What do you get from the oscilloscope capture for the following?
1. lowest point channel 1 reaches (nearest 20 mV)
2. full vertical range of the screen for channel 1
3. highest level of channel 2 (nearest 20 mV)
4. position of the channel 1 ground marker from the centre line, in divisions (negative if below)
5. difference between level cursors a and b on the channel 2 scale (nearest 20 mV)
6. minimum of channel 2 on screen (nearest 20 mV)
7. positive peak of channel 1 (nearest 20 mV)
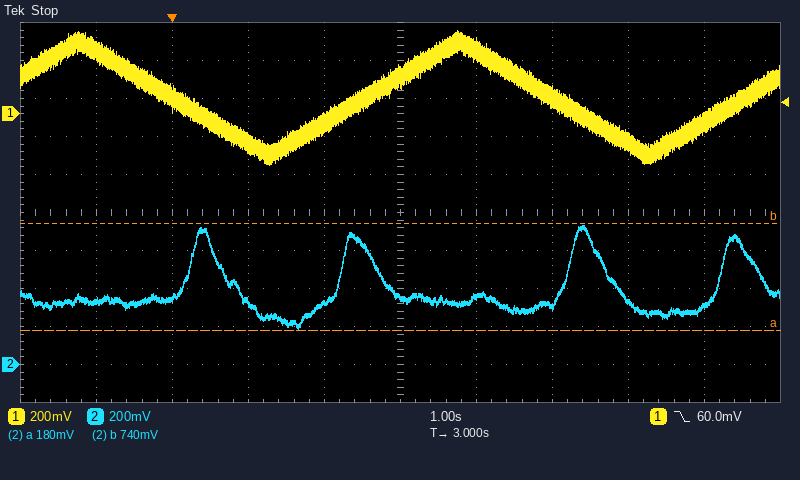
-280 mV
2 V
740 mV
+2.6 div
560 mV
180 mV
440 mV
